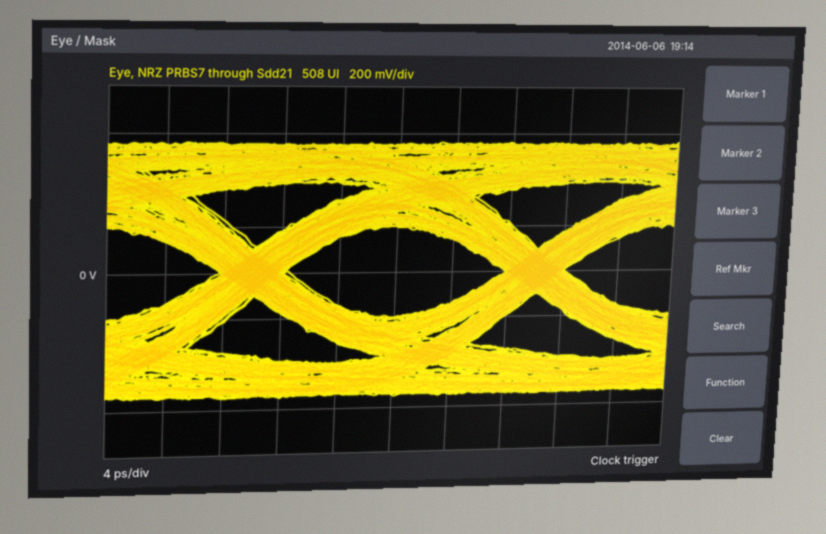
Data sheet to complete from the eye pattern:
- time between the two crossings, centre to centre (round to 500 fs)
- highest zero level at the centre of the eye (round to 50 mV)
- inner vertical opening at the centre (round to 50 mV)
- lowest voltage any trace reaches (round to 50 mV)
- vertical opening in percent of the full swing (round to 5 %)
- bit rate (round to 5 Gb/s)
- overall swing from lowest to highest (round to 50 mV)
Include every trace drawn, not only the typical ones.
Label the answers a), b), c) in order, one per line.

a) 20.0 ps
b) -200 mV
c) 400 mV
d) -550 mV
e) 35 %
f) 50 Gb/s
g) 1.10 V
